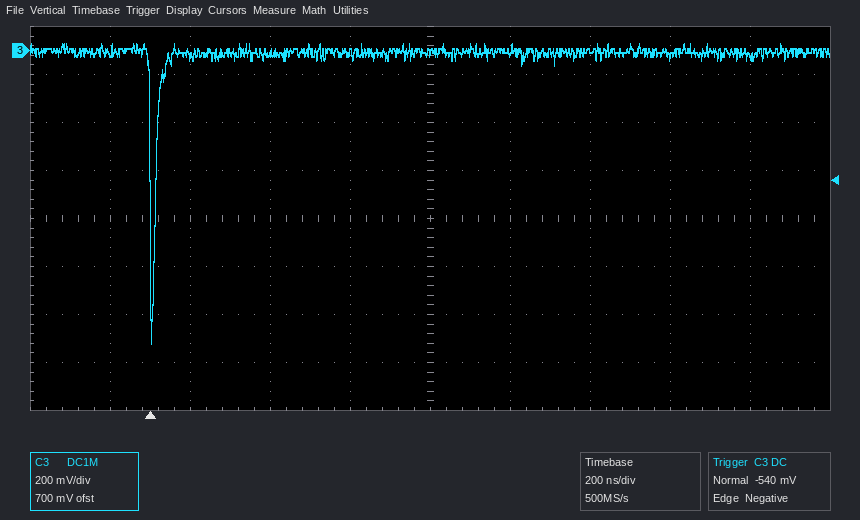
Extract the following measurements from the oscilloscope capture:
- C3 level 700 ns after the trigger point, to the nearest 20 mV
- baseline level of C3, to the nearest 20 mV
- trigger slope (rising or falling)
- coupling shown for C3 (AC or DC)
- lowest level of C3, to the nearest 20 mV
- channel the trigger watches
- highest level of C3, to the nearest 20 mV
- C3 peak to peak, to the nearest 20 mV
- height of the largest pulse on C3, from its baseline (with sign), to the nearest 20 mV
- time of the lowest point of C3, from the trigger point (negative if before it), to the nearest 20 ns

0 mV
0 mV
falling
DC
-1.22 V
C3
20 mV
1.24 V
-1.22 V
0 ns
